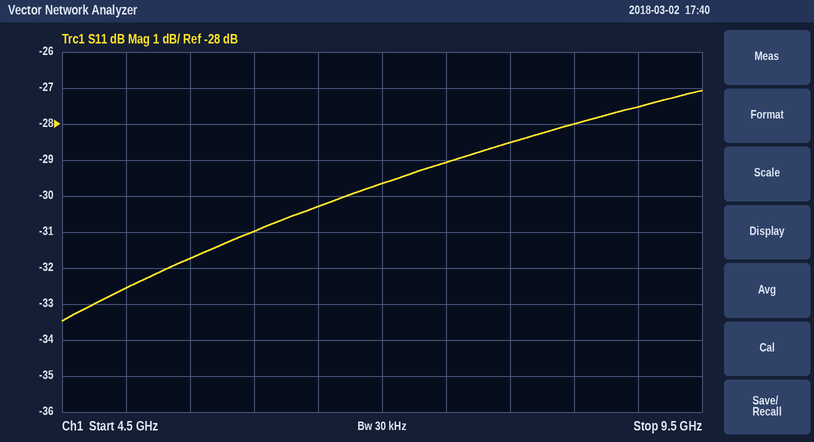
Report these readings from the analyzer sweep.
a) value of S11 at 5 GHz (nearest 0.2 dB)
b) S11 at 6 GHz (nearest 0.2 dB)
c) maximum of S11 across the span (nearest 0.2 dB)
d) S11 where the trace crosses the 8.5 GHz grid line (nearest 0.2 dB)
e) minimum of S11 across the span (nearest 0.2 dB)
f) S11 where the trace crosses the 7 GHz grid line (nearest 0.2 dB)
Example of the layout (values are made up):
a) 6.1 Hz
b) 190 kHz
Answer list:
a) -32.6 dB
b) -31.0 dB
c) -27.0 dB
d) -28.0 dB
e) -33.4 dB
f) -29.6 dB
